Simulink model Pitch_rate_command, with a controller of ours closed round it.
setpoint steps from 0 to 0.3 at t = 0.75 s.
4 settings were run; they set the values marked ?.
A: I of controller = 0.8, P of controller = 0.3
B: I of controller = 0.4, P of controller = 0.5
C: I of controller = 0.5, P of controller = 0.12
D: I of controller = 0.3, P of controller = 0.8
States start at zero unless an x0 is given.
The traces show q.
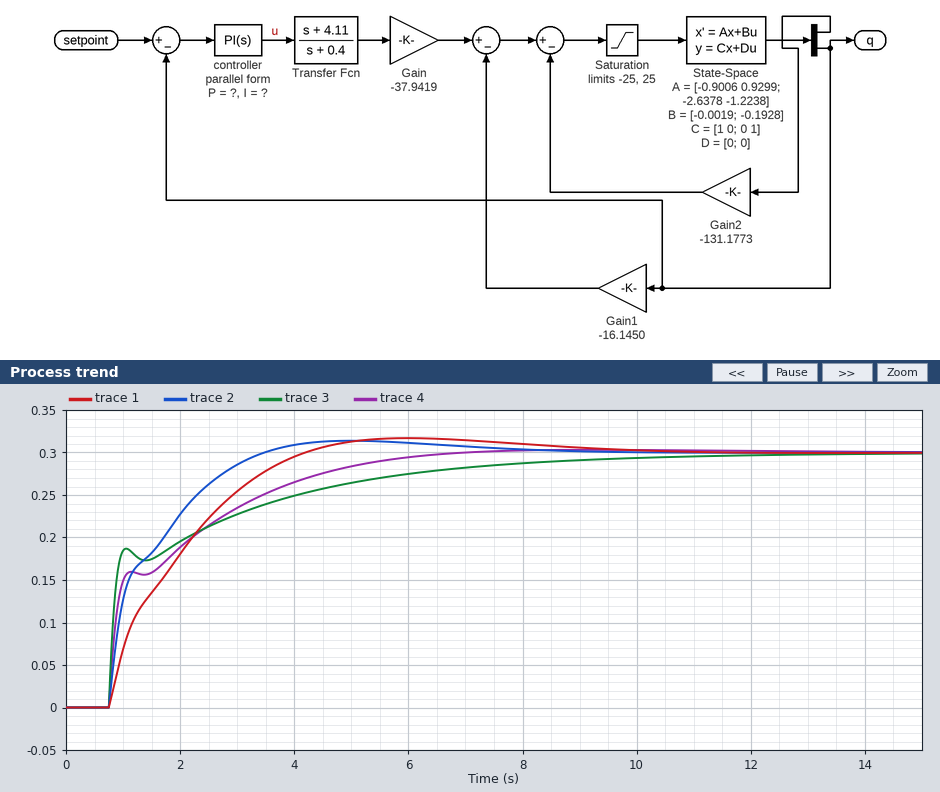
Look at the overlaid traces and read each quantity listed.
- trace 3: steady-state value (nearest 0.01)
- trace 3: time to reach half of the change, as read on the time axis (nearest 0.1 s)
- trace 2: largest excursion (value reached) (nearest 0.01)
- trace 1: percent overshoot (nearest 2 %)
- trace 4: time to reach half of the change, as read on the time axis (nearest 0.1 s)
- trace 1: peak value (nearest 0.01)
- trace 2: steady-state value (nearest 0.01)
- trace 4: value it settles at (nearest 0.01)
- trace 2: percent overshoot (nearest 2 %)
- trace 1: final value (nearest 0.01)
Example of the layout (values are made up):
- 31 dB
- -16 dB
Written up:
- 0.30
- 0.9 s
- 0.31
- 6 %
- 1.0 s
- 0.32
- 0.30
- 0.30
- 4 %
- 0.30
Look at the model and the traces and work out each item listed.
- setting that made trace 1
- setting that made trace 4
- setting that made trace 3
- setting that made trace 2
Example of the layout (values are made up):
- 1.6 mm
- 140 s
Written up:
- C
- B
- D
- A
